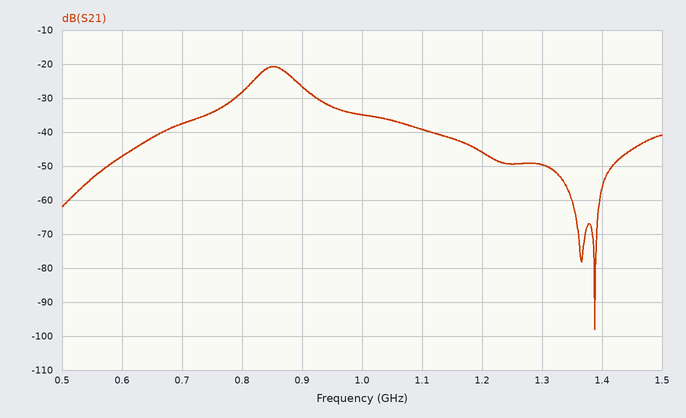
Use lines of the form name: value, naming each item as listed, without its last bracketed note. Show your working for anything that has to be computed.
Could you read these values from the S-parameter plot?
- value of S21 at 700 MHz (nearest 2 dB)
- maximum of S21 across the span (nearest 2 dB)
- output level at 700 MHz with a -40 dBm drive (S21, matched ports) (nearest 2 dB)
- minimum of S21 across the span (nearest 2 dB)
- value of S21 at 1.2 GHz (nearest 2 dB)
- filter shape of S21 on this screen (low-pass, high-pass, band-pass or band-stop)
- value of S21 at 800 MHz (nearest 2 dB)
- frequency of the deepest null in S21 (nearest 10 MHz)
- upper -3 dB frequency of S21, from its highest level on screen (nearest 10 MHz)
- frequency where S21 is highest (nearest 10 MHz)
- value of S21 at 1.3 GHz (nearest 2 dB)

value of S21 at 700 MHz: -38 dB
maximum of S21 across the span: -20 dB
output level at 700 MHz with a -40 dBm drive (S21, matched ports): -40 dBm + (-38 dB) = -78 dBm
minimum of S21 across the span: -98 dB
value of S21 at 1.2 GHz: -46 dB
filter shape of S21 on this screen: band-pass
value of S21 at 800 MHz: -28 dB
frequency of the deepest null in S21: 1.39 GHz
upper -3 dB frequency of S21, from its highest level on screen: 880 MHz
frequency where S21 is highest: 850 MHz
value of S21 at 1.3 GHz: -50 dB
